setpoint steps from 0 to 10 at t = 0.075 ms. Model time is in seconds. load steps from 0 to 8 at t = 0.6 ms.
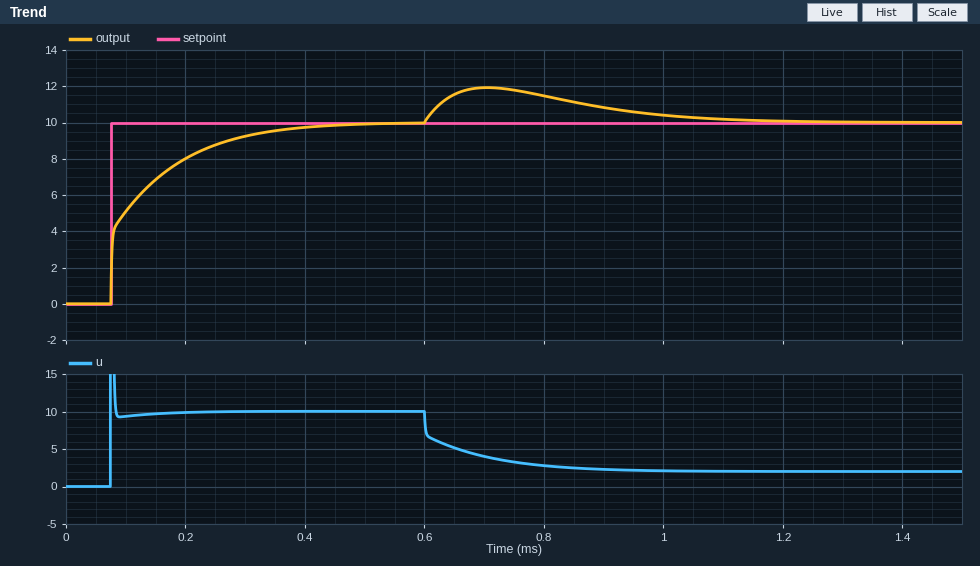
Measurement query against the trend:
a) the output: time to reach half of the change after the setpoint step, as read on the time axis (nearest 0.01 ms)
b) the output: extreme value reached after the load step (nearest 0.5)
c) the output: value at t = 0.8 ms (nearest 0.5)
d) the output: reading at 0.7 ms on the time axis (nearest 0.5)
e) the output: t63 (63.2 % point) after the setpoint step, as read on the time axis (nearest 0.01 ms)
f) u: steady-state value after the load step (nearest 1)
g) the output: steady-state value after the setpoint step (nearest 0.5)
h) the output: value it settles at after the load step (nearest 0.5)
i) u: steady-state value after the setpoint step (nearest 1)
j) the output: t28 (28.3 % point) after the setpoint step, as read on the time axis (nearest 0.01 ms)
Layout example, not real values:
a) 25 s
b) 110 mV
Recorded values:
a) 0.10 ms
b) 12.0
c) 11.5
d) 12.0
e) 0.13 ms
f) 2
g) 10.0
h) 10.0
i) 10
j) 0.08 ms
